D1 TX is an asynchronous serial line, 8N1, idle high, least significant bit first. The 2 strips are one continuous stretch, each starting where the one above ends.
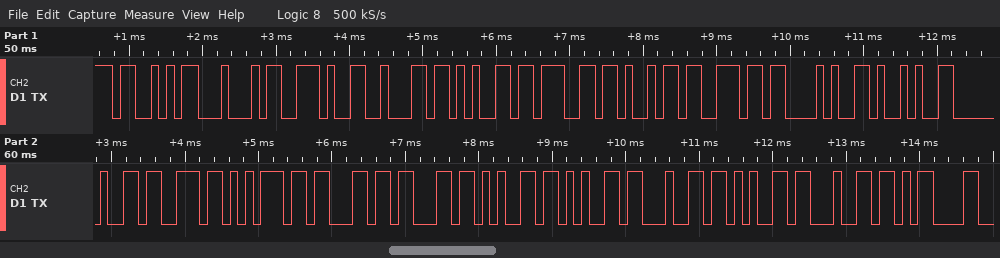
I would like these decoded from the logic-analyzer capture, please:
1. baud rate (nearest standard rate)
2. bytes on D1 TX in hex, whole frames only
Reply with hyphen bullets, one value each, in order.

- 9600 baud
- 53 44 2E 62 65 67 69 6E 28 29 20 73 75 63 63 65 65 64 65 64 0D
